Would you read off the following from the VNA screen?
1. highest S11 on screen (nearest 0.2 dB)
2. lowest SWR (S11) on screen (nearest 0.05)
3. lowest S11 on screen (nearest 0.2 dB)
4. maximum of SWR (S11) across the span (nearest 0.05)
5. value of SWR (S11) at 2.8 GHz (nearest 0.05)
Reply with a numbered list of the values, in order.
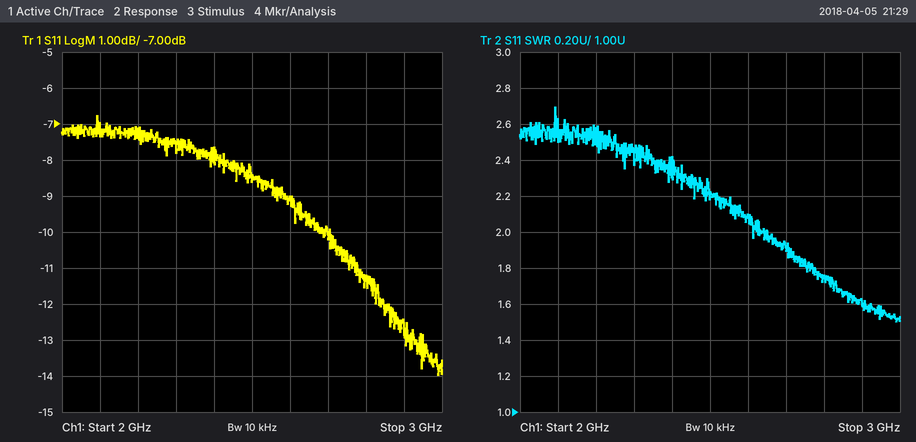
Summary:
1. -6.8 dB
2. 1.50
3. -14.0 dB
4. 2.70
5. 1.75
